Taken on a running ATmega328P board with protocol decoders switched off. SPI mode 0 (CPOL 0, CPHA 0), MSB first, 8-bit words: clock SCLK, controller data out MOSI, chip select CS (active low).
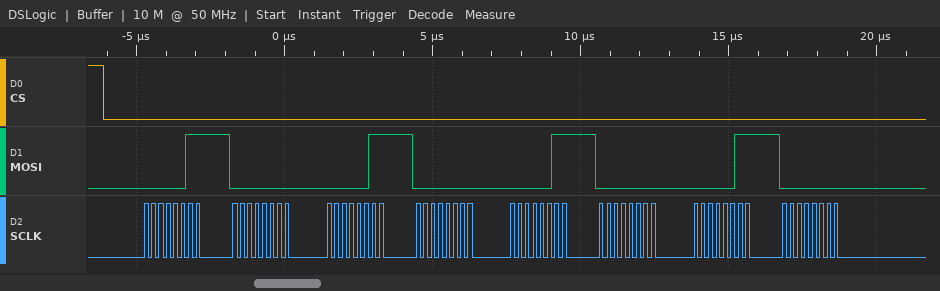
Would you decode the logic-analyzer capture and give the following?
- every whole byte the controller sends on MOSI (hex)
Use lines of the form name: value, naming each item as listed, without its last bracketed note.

every whole byte the controller sends on MOSI: 03 00 03 00 03 00 03 00
